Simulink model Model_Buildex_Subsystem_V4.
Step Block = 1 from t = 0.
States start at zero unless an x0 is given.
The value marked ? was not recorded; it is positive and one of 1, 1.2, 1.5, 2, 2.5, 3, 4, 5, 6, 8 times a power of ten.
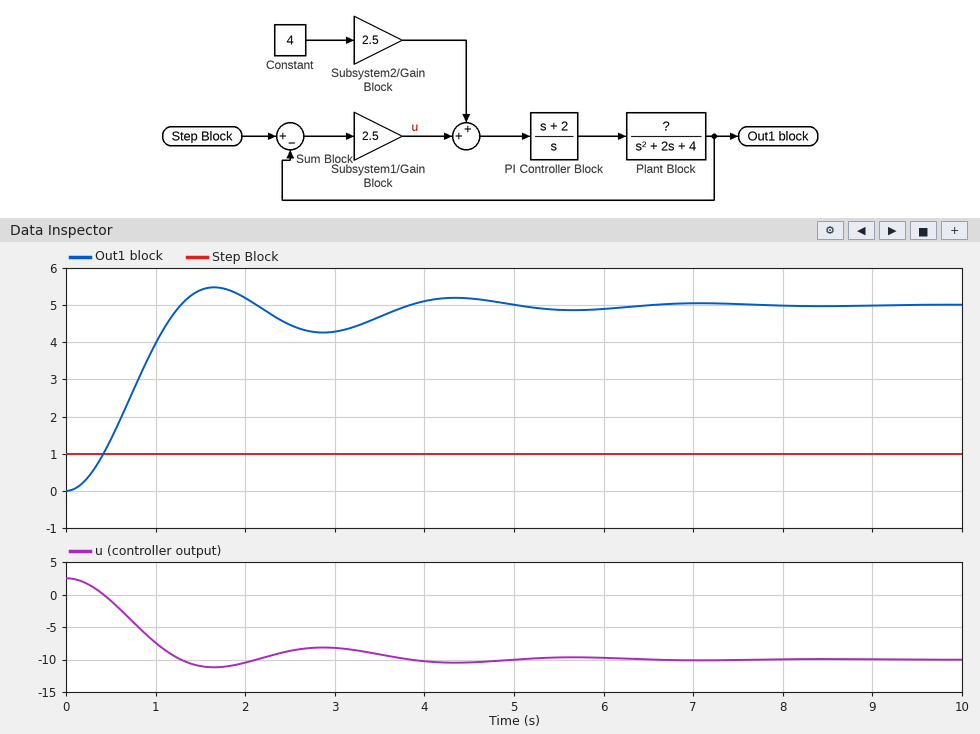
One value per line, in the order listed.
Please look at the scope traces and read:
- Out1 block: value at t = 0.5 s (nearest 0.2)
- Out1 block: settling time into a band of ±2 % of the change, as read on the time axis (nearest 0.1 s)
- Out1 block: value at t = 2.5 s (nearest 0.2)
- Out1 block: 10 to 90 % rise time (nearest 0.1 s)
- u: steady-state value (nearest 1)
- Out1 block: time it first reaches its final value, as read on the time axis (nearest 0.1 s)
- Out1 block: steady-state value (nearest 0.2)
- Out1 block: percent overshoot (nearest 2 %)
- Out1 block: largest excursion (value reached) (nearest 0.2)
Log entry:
1.4
6.0 s
4.4
0.8 s
-10
1.3 s
5.0
10 %
5.4
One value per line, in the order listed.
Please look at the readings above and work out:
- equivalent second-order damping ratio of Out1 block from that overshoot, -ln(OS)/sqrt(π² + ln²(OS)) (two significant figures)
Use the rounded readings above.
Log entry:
0.59
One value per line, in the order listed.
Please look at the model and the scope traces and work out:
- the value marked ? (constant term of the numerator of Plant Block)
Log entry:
1
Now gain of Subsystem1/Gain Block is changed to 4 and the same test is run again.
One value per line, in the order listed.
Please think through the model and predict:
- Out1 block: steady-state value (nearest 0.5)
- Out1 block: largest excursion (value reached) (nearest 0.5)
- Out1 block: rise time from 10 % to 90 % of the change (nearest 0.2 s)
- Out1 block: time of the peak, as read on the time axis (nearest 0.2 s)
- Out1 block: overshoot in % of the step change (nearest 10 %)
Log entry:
3.5
4.5
0.6 s
1.4 s
30 %
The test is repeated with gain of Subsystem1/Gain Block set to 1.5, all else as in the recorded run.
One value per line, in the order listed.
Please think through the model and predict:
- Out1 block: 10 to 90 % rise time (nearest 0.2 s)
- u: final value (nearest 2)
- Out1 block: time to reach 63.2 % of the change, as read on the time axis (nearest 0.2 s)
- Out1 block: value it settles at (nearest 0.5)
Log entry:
1.6 s
-10
1.2 s
7.5
